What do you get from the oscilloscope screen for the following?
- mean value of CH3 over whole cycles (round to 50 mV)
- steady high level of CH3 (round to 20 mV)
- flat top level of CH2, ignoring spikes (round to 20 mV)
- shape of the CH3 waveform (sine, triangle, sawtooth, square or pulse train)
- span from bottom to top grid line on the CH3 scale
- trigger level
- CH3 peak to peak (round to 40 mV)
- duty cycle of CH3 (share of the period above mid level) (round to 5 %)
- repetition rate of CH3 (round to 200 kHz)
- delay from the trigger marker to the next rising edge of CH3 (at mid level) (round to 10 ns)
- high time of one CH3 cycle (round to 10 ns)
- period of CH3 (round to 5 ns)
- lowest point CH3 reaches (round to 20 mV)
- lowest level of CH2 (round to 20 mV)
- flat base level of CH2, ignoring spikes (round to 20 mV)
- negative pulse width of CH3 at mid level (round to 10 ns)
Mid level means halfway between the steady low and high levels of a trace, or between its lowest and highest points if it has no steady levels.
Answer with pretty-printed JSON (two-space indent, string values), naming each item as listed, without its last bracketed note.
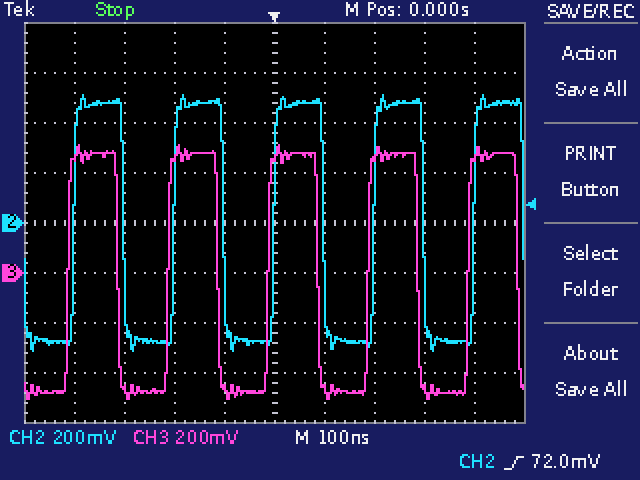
{
  "mean value of CH3 over whole cycles": "0 mV",
  "steady high level of CH3": "480 mV",
  "flat top level of CH2, ignoring spikes": "480 mV",
  "shape of the CH3 waveform": "square",
  "span from bottom to top grid line on the CH3 scale": "1.6 V",
  "trigger level": "72.0 mV",
  "CH3 peak to peak": "1.00 V",
  "duty cycle of CH3 (share of the period above mid level)": "50 %",
  "repetition rate of CH3": "5.0 MHz",
  "delay from the trigger marker to the next rising edge of CH3 (at mid level)": "190 ns",
  "high time of one CH3 cycle": "100 ns",
  "period of CH3": "200 ns",
  "lowest point CH3 reaches": "-500 mV",
  "lowest level of CH2": "-520 mV",
  "flat base level of CH2, ignoring spikes": "-480 mV",
  "negative pulse width of CH3 at mid level": "100 ns"
}
